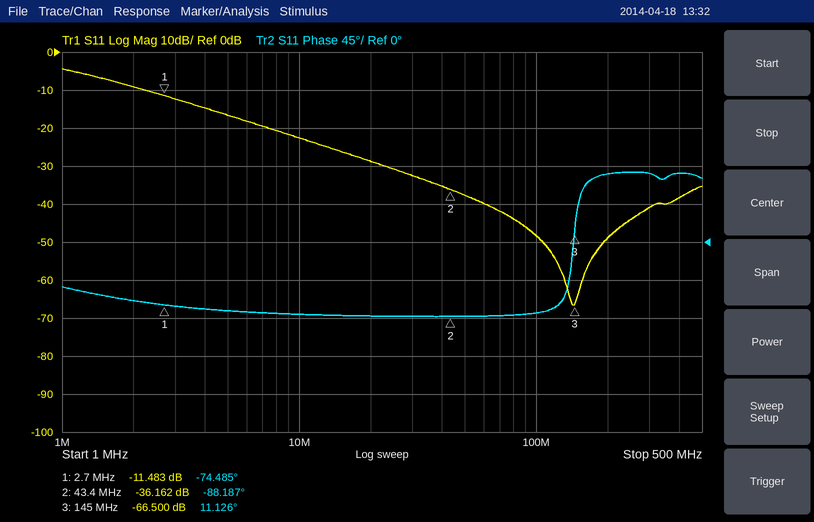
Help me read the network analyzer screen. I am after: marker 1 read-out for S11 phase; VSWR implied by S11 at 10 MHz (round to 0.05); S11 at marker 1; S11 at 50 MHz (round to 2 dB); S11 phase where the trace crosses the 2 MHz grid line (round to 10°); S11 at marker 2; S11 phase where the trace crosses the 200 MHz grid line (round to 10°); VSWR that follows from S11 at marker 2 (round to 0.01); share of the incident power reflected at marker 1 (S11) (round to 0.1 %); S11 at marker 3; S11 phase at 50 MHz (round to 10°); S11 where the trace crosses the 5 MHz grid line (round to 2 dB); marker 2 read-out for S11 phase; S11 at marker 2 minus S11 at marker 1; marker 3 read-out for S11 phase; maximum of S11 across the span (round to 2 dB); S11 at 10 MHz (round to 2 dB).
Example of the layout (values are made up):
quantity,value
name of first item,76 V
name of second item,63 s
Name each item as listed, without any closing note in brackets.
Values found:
quantity,value
marker 1 read-out for S11 phase,-74.485°
VSWR implied by S11 at 10 MHz,1.15
S11 at marker 1,-11.483 dB
S11 at 50 MHz,-38 dB
S11 phase where the trace crosses the 2 MHz grid line,-70°
S11 at marker 2,-36.162 dB
S11 phase where the trace crosses the 200 MHz grid line,80°
VSWR that follows from S11 at marker 2,1.03
share of the incident power reflected at marker 1 (S11),7.1 %
S11 at marker 3,-66.500 dB
S11 phase at 50 MHz,-90°
S11 where the trace crosses the 5 MHz grid line,-16 dB
marker 2 read-out for S11 phase,-88.187°
S11 at marker 2 minus S11 at marker 1,-24.679 dB
marker 3 read-out for S11 phase,11.126°
maximum of S11 across the span,-4 dB
S11 at 10 MHz,-22 dB
